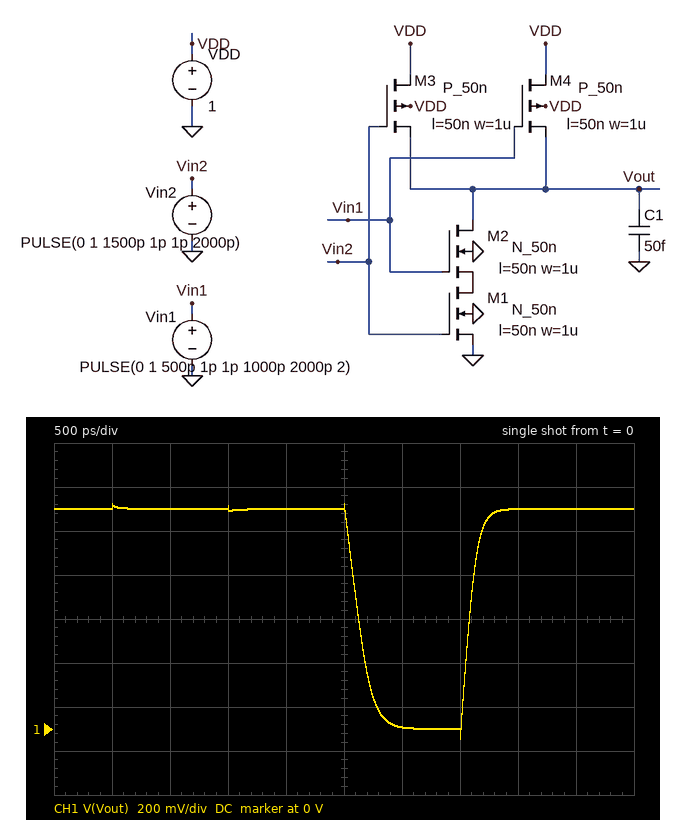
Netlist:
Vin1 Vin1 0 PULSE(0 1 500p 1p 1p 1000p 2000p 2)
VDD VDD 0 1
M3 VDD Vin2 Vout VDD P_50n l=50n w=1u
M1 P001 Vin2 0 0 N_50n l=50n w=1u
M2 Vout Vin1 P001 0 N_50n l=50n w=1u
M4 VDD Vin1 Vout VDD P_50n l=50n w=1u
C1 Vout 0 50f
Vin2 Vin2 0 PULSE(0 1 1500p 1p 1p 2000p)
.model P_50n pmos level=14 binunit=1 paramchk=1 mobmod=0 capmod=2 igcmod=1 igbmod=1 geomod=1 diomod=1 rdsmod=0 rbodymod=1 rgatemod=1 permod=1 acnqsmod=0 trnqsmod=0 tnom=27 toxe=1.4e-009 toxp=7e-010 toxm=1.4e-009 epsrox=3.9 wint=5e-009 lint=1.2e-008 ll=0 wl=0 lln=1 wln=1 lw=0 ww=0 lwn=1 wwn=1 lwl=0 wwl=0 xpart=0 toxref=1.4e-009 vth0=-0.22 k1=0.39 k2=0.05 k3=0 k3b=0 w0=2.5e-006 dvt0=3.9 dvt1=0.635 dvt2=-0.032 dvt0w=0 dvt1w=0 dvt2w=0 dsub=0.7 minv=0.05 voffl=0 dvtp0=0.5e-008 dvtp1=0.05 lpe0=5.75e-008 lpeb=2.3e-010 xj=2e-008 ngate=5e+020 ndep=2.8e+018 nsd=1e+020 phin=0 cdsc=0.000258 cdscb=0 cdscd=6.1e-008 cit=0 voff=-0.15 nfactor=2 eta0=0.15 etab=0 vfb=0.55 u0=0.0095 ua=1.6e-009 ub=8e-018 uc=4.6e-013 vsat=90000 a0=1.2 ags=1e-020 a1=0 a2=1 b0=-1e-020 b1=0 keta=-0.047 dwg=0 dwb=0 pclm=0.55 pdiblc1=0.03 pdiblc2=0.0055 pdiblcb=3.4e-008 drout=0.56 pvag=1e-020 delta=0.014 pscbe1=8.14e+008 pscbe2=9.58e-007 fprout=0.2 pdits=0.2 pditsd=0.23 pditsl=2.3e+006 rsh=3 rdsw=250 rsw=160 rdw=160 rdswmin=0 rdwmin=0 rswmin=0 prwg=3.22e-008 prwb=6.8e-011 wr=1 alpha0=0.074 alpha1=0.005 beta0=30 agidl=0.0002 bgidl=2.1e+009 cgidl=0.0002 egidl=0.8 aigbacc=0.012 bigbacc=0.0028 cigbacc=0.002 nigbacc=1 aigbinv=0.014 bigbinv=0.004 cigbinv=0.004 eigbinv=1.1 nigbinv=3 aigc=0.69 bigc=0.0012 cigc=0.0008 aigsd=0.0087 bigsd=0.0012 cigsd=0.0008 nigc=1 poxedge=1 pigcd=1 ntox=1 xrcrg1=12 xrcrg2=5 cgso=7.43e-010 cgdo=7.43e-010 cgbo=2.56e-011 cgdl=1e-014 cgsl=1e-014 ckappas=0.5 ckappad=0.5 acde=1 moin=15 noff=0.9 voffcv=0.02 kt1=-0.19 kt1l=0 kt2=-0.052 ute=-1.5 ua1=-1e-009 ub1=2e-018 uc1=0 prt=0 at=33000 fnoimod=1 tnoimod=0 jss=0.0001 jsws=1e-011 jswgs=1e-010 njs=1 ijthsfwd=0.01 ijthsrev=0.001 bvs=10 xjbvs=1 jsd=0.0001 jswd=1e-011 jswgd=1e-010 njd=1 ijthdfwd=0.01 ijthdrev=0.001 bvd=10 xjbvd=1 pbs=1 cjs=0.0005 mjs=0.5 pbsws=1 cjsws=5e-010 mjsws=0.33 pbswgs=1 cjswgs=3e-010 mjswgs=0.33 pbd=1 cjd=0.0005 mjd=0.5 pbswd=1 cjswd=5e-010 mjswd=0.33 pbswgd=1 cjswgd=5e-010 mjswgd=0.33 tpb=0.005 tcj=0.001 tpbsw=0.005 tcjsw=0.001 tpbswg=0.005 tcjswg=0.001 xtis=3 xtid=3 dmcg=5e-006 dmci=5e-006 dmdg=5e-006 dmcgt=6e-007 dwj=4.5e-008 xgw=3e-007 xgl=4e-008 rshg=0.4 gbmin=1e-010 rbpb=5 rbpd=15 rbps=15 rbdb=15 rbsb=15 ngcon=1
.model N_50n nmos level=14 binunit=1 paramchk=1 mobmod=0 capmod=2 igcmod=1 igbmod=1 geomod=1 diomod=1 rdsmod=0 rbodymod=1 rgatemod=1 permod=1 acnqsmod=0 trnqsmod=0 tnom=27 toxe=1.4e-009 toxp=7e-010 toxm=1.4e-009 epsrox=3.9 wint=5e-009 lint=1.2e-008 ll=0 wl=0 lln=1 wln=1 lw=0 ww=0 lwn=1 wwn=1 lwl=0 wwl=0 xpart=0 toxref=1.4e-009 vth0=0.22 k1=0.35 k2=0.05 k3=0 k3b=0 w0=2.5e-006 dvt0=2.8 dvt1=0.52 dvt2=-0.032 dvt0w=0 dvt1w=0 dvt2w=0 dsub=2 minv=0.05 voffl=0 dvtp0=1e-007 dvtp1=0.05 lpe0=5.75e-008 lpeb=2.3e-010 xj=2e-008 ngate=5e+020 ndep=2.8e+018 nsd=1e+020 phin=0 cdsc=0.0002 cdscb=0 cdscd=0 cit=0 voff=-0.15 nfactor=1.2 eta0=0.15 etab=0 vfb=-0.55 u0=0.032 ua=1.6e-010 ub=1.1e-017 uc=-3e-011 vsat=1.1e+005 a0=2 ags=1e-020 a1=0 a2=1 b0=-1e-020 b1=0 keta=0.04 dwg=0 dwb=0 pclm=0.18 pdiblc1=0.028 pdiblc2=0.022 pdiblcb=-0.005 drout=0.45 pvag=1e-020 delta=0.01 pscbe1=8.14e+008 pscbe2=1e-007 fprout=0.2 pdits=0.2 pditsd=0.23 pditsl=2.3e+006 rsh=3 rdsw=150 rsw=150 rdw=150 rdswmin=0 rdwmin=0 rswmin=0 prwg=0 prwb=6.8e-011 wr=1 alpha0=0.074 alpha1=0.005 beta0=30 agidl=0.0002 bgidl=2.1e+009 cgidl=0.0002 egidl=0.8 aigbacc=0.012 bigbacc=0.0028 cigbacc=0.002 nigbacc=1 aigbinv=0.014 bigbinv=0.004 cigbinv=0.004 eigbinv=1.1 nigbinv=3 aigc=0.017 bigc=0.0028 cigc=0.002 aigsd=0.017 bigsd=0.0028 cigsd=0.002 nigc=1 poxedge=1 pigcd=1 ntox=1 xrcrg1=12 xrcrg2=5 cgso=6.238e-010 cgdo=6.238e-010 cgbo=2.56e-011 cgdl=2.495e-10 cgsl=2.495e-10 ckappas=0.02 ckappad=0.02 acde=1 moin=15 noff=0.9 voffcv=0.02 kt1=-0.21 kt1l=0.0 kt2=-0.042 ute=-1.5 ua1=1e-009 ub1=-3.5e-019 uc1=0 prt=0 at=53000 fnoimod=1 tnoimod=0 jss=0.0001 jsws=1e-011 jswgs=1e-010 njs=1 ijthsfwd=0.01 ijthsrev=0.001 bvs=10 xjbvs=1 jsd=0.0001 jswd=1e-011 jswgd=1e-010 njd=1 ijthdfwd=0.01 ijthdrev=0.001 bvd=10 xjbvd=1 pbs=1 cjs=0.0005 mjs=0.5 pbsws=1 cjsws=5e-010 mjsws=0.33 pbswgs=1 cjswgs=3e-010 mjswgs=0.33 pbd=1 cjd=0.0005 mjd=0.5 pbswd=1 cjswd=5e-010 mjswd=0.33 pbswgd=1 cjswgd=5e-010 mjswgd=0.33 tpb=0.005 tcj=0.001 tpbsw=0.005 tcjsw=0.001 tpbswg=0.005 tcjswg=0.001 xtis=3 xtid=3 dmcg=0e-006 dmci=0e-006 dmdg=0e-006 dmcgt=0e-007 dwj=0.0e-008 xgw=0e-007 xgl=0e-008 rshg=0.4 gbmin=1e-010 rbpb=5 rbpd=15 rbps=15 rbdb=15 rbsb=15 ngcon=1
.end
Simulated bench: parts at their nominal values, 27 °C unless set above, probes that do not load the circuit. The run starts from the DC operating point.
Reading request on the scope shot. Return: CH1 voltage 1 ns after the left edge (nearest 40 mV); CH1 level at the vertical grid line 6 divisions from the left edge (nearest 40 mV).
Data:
1.00 V
0 V
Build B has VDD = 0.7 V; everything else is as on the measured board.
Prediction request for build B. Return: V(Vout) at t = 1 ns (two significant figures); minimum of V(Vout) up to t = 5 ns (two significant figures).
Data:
700 mV
-43 mV
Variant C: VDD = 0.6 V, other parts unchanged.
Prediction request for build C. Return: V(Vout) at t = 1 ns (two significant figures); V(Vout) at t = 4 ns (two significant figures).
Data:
600 mV
590 mV
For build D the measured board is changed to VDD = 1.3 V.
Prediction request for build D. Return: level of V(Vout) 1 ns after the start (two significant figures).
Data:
1.3 V
